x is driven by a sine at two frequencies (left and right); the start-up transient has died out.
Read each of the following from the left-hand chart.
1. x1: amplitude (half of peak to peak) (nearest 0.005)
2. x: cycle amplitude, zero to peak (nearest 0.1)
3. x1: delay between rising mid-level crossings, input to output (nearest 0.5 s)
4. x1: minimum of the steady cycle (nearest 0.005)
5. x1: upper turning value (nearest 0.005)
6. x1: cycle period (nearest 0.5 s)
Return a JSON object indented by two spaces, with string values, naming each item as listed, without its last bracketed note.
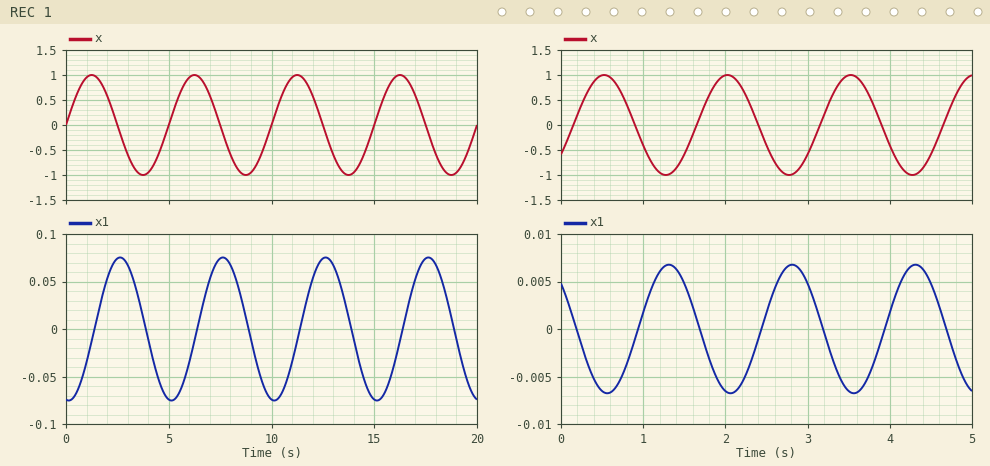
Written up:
{
  "x1: amplitude (half of peak to peak)": "0.075",
  "x: cycle amplitude, zero to peak": "1.0",
  "x1: delay between rising mid-level crossings, input to output": "1.5 s",
  "x1: minimum of the steady cycle": "-0.075",
  "x1: upper turning value": "0.075",
  "x1: cycle period": "5.0 s"
}
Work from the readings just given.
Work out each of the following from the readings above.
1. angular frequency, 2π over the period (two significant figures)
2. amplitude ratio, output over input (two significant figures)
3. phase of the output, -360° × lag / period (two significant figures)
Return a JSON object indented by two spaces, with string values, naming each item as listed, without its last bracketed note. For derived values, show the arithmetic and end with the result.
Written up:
{
  "angular frequency, 2π over the period": "2π / 5 = 1.3 rad/s",
  "amplitude ratio, output over input": "0.075 / 1 = 0.075",
  "phase of the output, -360° × lag / period": "-360 × 1.5 / 5 = -110°"
}
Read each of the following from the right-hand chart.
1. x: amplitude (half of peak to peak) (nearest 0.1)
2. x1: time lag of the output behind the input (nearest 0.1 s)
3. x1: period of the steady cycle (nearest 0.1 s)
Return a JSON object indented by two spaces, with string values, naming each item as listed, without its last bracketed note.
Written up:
{
  "x: amplitude (half of peak to peak)": "1.0",
  "x1: time lag of the output behind the input": "0.8 s",
  "x1: period of the steady cycle": "1.5 s"
}
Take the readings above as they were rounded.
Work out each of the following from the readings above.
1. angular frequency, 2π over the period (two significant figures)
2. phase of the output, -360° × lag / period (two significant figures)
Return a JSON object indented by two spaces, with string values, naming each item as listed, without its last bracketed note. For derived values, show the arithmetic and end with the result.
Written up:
{
  "angular frequency, 2π over the period": "2π / 1.5 = 4.2 rad/s",
  "phase of the output, -360° × lag / period": "-360 × 0.8 / 1.5 = -190°"
}
